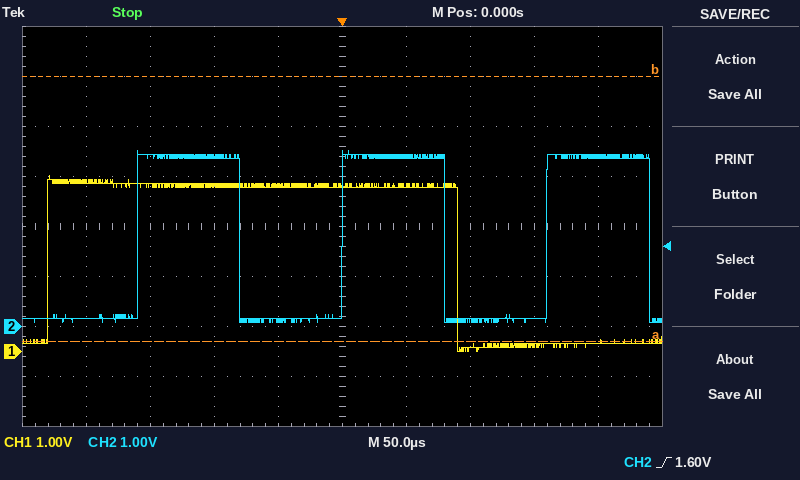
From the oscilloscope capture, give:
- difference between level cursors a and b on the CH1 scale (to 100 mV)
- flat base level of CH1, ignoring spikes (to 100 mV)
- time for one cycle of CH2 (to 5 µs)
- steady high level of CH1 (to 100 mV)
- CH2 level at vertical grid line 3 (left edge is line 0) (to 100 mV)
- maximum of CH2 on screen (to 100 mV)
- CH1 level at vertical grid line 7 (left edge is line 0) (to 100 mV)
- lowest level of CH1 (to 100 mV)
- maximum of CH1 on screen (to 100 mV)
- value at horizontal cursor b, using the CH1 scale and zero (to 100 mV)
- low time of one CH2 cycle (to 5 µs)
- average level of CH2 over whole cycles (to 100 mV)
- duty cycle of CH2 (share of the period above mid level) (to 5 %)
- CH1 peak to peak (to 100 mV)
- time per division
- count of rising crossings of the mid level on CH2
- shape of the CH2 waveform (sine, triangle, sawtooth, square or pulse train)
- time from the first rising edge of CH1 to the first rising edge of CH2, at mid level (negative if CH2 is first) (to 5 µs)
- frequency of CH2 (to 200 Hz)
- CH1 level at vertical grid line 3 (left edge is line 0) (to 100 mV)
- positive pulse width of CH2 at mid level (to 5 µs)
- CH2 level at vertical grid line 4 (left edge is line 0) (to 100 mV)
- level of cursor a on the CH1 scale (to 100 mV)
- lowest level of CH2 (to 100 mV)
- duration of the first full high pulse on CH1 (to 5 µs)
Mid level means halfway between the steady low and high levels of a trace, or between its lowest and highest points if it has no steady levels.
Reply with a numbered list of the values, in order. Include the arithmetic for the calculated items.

1. 5.3 V
2. 200 mV
3. 160 µs
4. 3.3 V
5. 3.4 V
6. 3.5 V
7. 0.0 V
8. 0.0 V
9. 3.5 V
10. 5.5 V
11. 80 µs
12. 100 mV + 0.5 × (3.5 V − (100 mV)) ≈ 1.8 V
13. 80 µs / 160 µs ≈ 50 %
14. 3.5 V − (0.0 V) = 3.5 V
15. 50 µs
16. 3
17. square
18. +70 µs
19. 1 / 160 µs ≈ 6.2 kHz
20. 3.3 V
21. 80 µs
22. 100 mV
23. 200 mV
24. 100 mV
25. 320 µs
